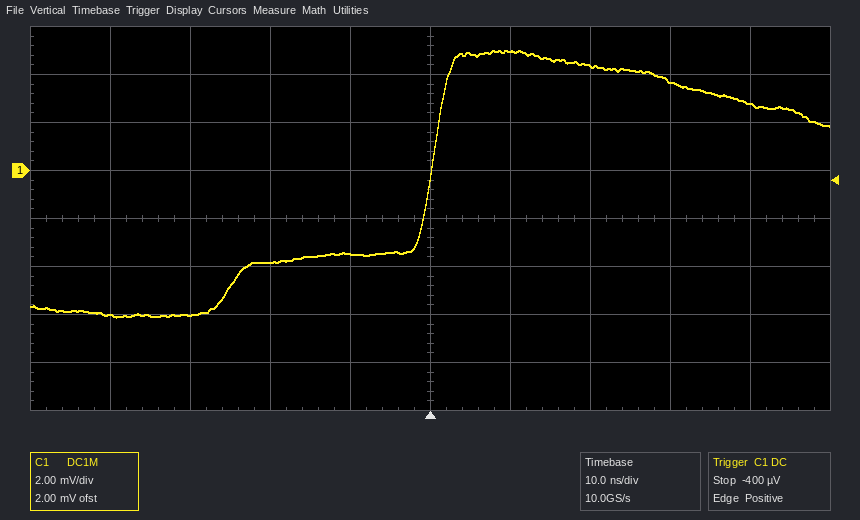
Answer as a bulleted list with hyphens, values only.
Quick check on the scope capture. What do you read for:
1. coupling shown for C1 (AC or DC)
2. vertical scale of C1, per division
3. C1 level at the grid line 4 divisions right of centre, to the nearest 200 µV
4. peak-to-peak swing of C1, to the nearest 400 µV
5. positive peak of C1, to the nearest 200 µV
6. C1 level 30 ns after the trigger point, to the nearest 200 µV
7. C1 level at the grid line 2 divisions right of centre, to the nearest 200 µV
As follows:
- DC
- 2 mV
- 2.8 mV
- 11.2 mV
- 5.0 mV
- 3.8 mV
- 4.4 mV
